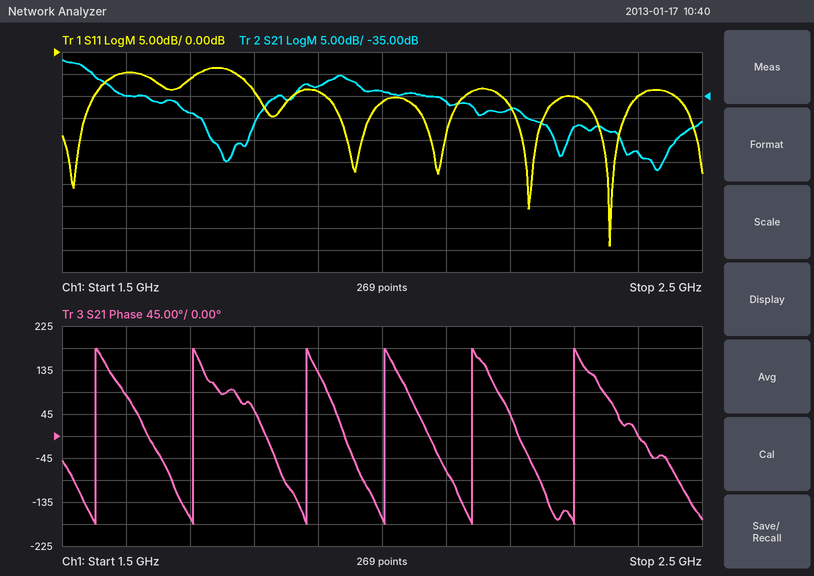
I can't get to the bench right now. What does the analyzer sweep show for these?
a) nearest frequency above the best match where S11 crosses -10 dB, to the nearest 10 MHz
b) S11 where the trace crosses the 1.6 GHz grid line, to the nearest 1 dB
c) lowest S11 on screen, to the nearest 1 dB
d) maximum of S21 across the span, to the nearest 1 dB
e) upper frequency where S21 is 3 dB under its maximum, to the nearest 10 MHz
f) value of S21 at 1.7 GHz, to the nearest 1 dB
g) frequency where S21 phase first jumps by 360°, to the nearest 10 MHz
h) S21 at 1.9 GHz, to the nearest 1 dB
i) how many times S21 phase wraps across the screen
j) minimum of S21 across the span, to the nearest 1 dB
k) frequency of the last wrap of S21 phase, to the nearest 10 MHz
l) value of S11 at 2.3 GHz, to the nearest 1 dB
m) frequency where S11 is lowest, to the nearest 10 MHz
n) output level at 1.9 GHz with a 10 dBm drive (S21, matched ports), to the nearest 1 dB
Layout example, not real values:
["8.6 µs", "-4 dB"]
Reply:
["2.40 GHz", "-5 dB", "-44 dB", "-27 dB", "1.55 GHz", "-39 dB", "1.55 GHz", "-33 dB", "6", "-52 dB", "2.30 GHz", "-10 dB", "2.36 GHz", "-23 dBm"]
